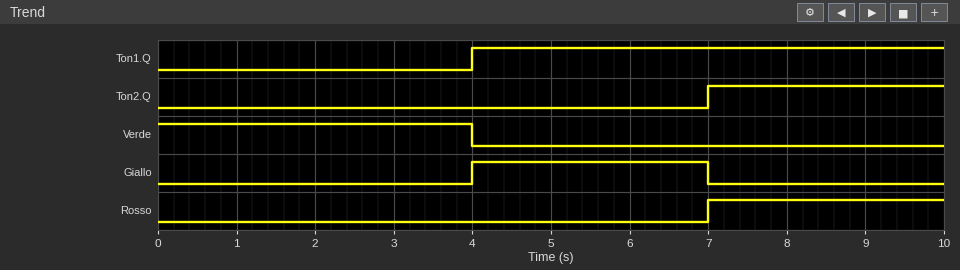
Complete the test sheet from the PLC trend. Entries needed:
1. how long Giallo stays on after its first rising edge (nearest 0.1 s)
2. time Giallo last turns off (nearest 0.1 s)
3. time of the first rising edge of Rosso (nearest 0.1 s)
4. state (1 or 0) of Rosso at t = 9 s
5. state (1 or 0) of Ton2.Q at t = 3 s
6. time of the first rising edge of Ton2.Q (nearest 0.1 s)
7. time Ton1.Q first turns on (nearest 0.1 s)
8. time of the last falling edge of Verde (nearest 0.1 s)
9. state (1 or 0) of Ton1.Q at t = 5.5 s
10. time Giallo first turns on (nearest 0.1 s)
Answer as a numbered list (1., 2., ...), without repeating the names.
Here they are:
1. 3.0 s
2. 7.0 s
3. 7.0 s
4. 1
5. 0
6. 7.0 s
7. 4.0 s
8. 4.0 s
9. 1
10. 4.0 s
